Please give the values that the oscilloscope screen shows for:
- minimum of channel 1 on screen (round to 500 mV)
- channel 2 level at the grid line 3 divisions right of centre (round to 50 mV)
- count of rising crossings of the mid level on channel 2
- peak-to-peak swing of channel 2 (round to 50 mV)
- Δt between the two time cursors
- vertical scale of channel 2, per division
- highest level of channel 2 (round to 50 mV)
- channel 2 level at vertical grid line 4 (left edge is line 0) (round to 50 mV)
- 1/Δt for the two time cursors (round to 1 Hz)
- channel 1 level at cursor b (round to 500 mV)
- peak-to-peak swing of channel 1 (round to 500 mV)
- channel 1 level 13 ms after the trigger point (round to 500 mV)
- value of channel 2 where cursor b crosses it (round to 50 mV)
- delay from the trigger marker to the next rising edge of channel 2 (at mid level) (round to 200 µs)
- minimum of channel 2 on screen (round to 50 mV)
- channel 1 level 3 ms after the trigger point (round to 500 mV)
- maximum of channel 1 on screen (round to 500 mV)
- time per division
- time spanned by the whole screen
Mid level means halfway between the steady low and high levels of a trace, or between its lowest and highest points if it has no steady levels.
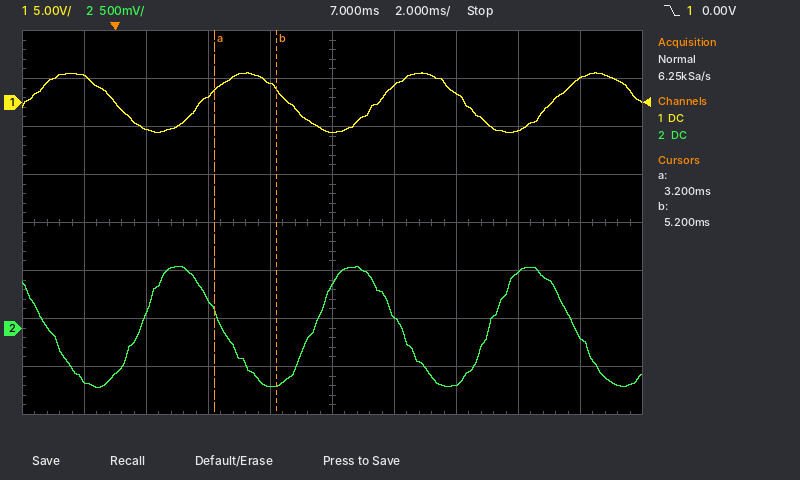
-3.0 V
600 mV
3
1.25 V
2.0 ms
500 mV
650 mV
-600 mV
500 Hz
1.5 V
6.0 V
-3.0 V
-600 mV
800 µs
-600 mV
500 mV
3.0 V
2 ms
20 ms
